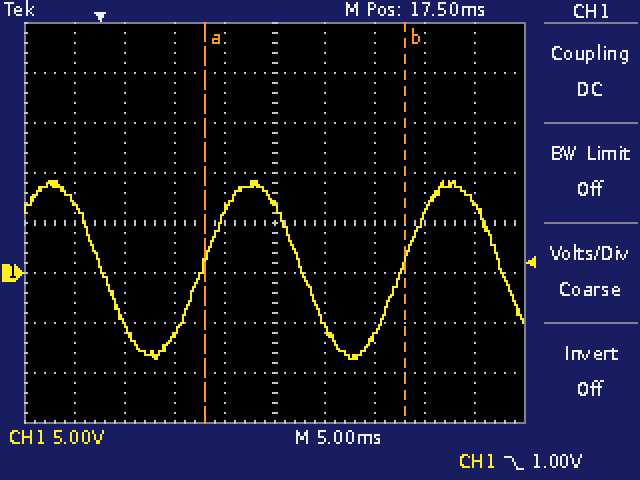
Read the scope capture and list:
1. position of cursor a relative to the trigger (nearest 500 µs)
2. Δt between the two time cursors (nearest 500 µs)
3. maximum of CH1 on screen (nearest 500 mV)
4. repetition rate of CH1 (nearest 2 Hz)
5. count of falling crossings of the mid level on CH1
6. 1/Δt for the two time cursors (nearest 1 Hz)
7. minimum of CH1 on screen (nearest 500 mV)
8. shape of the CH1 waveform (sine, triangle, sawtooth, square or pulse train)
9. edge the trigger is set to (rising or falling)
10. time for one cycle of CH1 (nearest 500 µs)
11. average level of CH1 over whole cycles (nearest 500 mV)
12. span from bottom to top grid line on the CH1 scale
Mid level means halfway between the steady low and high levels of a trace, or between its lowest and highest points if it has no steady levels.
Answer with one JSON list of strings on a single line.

["+10.5 ms", "20.0 ms", "9.0 V", "50 Hz", "3", "50 Hz", "-8.5 V", "sine", "falling", "20.0 ms", "500 mV", "40 V"]
